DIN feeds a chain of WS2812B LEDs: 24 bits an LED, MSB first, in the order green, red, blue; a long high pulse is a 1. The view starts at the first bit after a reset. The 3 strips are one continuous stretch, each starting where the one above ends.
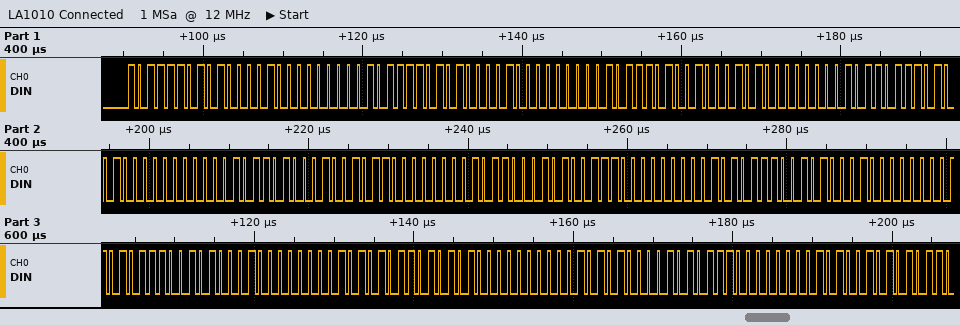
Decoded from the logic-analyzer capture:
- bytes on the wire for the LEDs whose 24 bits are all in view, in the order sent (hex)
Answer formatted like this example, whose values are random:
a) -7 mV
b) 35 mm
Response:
a) BD 42 00 BD 42 00 BA 45 00 B7 48 00 B4 4B 00 B1 4E 00 AE 51 00 AE 51 00 AB 54 00 A8 57 00
